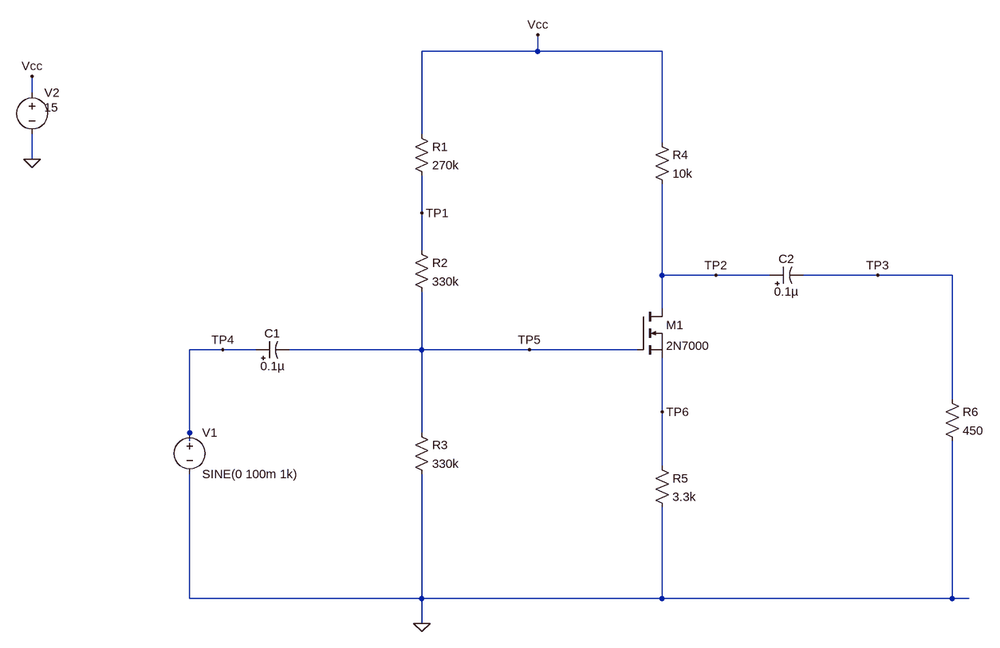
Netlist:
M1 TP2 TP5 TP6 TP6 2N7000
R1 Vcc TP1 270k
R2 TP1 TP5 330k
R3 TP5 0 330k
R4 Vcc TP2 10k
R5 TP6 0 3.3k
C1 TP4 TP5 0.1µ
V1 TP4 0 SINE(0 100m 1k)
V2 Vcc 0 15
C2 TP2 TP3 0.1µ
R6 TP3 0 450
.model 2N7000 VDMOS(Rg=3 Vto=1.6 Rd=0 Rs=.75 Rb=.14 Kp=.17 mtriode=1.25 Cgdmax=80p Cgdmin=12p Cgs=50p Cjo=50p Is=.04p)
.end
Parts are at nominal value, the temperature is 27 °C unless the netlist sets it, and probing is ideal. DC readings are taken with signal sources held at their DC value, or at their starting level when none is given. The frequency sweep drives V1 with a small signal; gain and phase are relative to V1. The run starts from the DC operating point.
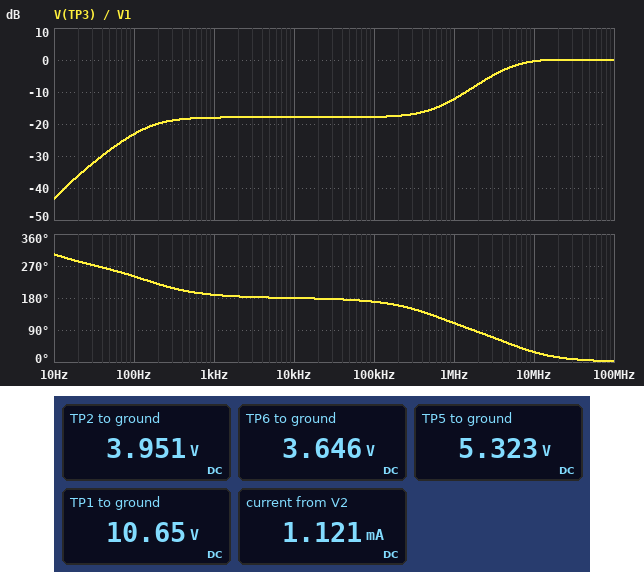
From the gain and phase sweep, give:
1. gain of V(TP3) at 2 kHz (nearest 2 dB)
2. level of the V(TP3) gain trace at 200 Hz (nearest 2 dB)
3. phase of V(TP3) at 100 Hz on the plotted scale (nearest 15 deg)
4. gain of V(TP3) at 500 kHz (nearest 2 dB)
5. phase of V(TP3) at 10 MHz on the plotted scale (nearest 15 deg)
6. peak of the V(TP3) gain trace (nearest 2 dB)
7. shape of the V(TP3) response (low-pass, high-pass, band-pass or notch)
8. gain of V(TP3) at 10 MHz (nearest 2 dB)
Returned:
-18 dB
-20 dB
240 deg
-16 dB
30 deg
0 dB
high-pass
0 dB
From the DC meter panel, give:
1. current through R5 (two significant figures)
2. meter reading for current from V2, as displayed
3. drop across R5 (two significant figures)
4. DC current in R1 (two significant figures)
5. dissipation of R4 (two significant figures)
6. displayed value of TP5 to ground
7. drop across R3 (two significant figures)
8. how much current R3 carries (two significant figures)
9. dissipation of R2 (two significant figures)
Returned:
1.1 mA
1.121 mA
3.6 V
16 µA
12 mW
5.323 V
5.3 V
16 µA
86 µW
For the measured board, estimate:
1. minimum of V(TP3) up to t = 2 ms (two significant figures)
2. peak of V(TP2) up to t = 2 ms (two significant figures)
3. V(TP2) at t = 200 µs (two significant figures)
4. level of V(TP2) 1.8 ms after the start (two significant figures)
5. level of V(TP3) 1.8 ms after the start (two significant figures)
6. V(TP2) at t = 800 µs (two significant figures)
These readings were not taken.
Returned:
-12 mV
4.0 V
3.9 V
4.0 V
12 mV
4.0 V
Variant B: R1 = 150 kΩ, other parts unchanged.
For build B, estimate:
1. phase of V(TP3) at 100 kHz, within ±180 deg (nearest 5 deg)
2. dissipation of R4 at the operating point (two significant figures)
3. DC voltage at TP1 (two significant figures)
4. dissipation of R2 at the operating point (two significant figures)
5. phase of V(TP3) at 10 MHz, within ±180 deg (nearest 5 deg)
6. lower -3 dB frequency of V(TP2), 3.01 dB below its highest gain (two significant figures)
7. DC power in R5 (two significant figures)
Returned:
90 deg
13 mW
12 V
110 µW
20 deg
3.2 MHz
4.2 mW
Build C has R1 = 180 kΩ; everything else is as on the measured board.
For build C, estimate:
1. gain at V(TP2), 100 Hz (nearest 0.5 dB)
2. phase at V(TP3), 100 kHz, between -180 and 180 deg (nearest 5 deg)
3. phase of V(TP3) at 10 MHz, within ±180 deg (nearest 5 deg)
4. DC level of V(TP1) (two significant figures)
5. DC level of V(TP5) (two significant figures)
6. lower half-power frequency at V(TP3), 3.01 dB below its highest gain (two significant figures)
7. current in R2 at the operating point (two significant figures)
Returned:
-38.5 dB
90 deg
20 deg
12 V
5.9 V
3.2 MHz
18 µA
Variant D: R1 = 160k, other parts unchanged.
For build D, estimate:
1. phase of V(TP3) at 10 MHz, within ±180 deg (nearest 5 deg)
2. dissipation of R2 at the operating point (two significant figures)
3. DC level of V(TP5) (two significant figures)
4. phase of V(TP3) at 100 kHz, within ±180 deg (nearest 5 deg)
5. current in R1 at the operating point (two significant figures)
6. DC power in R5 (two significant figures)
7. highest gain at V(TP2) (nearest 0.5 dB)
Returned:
20 deg
110 µW
6.0 V
90 deg
18 µA
4.2 mW
0 dB
